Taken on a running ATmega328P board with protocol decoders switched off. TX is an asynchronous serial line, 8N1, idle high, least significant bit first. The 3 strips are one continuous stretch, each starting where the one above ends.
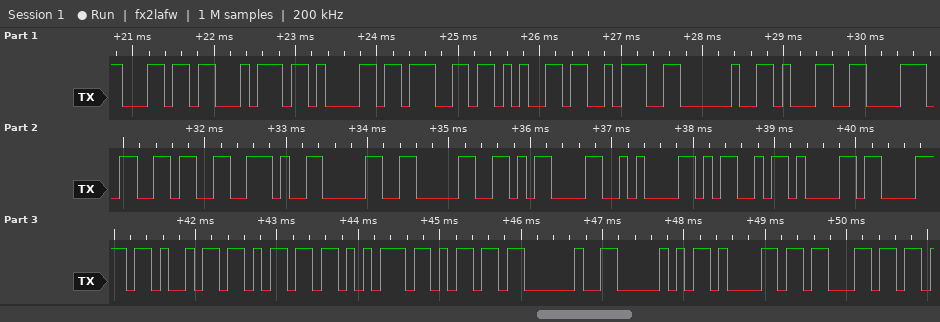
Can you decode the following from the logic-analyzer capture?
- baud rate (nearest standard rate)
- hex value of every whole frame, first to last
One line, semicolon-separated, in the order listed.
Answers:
9600 baud; 6C 74 61 67 65 3A 20 31 38 36 2E 30 30 0D 0A 4D 61 78 69 6D 75 6D 20 50 61 63
